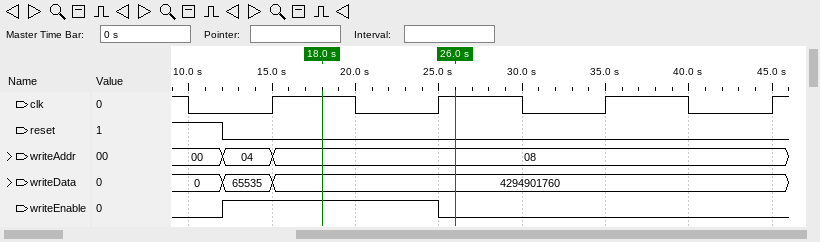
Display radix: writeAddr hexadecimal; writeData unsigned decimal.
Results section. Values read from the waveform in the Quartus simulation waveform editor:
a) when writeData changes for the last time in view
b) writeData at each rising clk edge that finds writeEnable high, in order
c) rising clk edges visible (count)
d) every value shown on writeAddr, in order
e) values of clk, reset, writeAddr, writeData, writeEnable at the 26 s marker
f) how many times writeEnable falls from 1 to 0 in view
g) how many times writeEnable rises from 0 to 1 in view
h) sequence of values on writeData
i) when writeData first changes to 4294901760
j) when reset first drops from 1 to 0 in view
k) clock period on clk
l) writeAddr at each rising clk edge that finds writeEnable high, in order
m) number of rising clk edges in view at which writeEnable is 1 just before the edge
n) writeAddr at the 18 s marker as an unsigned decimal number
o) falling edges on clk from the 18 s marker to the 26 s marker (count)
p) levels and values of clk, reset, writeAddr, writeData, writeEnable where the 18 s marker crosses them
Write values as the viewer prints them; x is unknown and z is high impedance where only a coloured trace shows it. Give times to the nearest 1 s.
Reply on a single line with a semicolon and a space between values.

15 s; 65535, 4294901760; 4; 00, 04, 08; clk=1, reset=0, writeAddr=08, writeData=4294901760, writeEnable=0; 1; 1; 0, 65535, 4294901760; 15 s; 12 s; 10 s; 04, 08; 2; 8; 1; clk=1, reset=0, writeAddr=08, writeData=4294901760, writeEnable=1
